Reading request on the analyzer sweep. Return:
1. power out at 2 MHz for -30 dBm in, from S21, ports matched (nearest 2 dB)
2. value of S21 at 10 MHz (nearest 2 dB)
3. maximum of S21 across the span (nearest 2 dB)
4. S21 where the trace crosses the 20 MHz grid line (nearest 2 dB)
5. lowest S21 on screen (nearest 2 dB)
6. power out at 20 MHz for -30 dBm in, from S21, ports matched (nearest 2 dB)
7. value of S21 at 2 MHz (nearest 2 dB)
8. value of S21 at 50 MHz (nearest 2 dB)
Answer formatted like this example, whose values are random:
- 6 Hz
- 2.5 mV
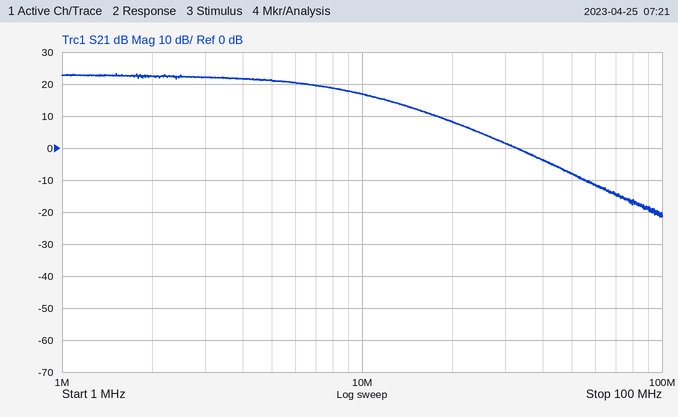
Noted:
- -8 dBm
- 16 dB
- 24 dB
- 8 dB
- -22 dB
- -22 dBm
- 22 dB
- -8 dB
